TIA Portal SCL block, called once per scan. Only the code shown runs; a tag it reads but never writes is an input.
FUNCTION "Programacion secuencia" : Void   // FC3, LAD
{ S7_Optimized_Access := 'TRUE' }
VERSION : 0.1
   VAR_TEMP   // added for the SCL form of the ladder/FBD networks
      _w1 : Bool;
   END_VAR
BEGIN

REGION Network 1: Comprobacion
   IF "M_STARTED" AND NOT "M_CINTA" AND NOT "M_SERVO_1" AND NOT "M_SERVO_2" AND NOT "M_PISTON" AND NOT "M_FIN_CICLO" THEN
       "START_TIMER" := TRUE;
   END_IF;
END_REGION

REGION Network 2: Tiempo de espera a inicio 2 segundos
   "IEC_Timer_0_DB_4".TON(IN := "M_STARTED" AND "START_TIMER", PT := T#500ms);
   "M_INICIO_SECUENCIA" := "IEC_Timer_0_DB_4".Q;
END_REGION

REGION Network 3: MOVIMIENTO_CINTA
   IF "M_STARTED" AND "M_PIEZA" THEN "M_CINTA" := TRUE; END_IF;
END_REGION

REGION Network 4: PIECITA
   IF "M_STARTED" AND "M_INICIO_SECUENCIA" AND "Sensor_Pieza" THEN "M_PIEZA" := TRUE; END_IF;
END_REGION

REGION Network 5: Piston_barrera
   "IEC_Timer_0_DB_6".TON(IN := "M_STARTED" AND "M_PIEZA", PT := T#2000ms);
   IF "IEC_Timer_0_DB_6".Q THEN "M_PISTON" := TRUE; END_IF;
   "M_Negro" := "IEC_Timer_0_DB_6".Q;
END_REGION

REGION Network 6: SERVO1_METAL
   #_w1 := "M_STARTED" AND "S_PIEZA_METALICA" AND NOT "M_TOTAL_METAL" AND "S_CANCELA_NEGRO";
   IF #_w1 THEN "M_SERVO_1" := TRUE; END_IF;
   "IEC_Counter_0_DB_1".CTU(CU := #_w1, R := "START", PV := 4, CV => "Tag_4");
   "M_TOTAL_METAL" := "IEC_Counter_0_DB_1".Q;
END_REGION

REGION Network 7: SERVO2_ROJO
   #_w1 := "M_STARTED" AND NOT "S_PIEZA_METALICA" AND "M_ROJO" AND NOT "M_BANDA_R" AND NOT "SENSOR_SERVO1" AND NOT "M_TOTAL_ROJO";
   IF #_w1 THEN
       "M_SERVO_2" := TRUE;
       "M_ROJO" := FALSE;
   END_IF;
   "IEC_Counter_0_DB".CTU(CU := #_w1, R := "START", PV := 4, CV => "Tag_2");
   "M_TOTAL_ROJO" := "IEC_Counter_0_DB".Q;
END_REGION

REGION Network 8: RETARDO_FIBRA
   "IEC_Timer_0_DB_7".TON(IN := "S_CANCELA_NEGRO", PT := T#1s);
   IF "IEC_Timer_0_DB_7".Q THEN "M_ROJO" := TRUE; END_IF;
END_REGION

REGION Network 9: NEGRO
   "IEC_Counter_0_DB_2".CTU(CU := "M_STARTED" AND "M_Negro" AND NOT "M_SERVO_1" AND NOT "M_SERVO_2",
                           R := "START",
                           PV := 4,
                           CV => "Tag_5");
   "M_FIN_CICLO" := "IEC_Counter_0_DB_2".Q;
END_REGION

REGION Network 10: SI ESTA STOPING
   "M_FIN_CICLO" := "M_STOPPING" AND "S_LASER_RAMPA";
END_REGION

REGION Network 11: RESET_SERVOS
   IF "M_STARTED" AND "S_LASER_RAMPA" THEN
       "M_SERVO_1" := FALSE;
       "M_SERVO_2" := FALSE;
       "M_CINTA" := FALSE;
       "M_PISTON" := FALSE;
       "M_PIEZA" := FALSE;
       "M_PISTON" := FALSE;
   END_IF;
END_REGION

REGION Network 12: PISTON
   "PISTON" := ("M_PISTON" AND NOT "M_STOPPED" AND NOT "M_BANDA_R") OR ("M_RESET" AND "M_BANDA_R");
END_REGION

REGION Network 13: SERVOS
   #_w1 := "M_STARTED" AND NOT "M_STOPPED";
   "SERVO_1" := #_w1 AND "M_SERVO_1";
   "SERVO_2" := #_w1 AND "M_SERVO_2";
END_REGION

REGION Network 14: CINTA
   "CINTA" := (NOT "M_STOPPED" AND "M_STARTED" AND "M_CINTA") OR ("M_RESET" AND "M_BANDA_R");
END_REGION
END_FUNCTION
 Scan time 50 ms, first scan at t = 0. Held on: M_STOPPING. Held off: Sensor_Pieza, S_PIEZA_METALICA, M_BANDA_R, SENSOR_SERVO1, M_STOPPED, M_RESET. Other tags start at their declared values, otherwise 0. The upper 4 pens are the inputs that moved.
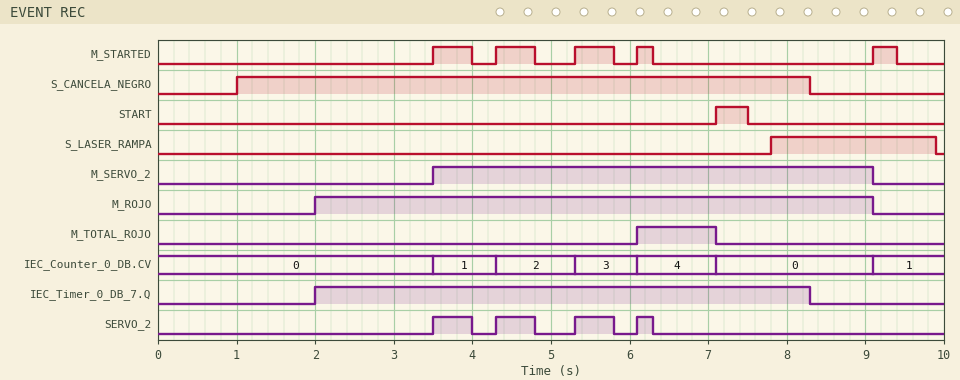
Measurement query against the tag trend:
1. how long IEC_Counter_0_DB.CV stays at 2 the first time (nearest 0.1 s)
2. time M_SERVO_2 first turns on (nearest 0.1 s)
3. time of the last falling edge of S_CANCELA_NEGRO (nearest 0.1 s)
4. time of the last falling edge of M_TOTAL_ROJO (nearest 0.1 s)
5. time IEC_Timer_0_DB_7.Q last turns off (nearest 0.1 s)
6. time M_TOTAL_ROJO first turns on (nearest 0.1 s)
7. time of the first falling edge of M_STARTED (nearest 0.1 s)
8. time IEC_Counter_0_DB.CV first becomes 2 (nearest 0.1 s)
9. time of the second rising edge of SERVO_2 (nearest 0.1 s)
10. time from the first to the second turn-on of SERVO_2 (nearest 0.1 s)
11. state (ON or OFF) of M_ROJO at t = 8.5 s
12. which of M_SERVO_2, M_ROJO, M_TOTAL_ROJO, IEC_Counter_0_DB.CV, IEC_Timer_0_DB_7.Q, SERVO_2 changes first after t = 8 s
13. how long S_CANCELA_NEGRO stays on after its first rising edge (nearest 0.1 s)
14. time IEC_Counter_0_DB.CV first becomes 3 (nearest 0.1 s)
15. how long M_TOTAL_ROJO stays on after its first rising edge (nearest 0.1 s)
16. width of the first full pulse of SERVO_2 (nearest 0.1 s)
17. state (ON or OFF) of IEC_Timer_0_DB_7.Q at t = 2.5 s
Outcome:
1.0 s
3.5 s
8.3 s
7.1 s
8.3 s
6.1 s
4.0 s
4.3 s
4.3 s
0.8 s
ON
IEC_Timer_0_DB_7.Q
7.3 s
5.3 s
1.0 s
0.5 s
ON
